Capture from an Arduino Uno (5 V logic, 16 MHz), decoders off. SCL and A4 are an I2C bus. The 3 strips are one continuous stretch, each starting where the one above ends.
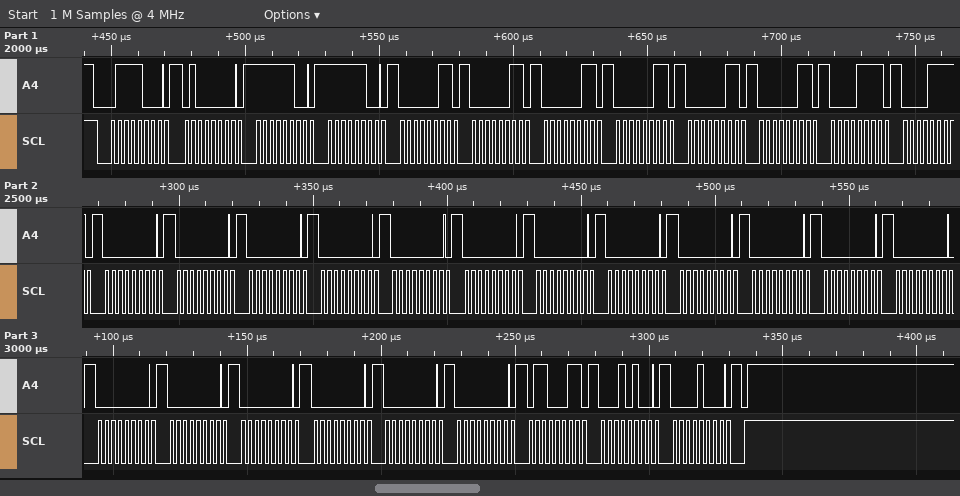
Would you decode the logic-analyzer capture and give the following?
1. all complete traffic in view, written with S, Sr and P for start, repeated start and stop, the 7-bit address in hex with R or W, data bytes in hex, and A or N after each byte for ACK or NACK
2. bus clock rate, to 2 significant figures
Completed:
S 3CW A 40 A FC A FC A 03 A 03 A 03 A 03 A 03 A 03 A 0F A 0F A 00 A 00 A 00 A 00 A 00 A 00 A 00 A 00 A 00 A 00 A 00 A 00 A 00 A 00 A 00 A 00 A 00 A 00 A 63 A 14 A 08 A P
400 kHz
